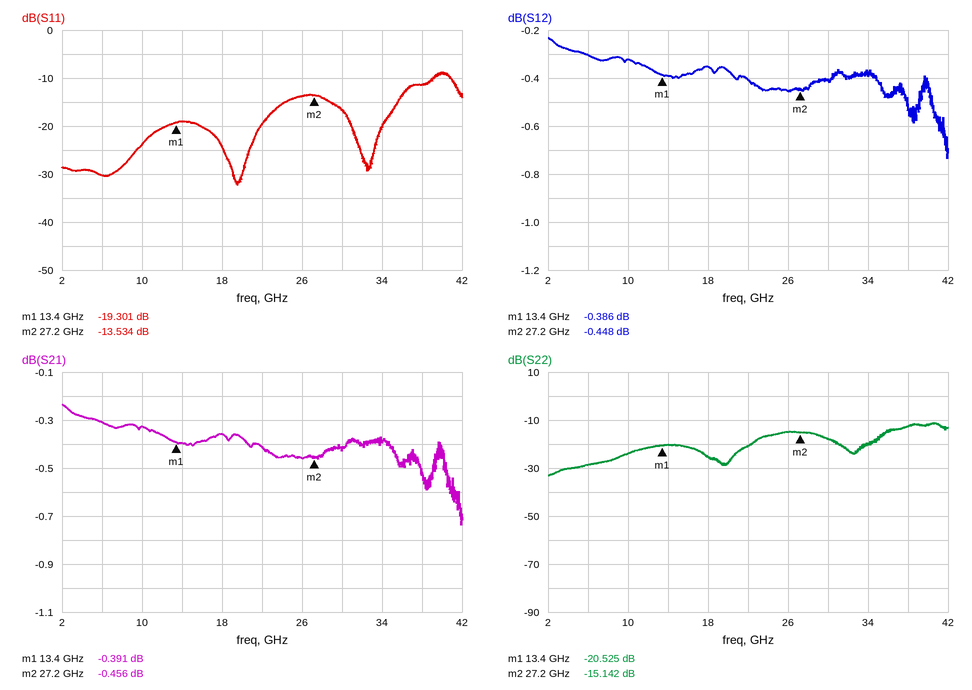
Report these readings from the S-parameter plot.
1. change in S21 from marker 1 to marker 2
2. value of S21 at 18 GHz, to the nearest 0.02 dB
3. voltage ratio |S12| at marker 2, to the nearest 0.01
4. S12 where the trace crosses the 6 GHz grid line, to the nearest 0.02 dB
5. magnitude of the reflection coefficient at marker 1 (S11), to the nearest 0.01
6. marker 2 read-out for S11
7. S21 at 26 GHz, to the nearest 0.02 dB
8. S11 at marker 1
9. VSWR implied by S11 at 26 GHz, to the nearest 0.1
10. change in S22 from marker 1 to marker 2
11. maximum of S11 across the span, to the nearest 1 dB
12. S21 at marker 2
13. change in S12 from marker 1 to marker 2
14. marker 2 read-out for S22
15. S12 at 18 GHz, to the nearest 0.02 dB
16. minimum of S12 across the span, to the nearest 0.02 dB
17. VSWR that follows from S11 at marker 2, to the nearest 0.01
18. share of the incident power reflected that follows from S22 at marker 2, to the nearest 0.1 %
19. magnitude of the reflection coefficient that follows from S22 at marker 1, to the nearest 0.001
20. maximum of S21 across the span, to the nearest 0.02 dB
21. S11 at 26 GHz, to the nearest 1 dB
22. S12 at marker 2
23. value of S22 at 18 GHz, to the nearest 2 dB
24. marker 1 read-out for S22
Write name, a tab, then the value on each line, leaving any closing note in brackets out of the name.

change in S21 from marker 1 to marker 2	-0.065 dB
value of S21 at 18 GHz, to the nearest 0.02 dB	-0.36 dB
voltage ratio |S12| at marker 2, to the nearest 0.01	0.95
S12 where the trace crosses the 6 GHz grid line, to the nearest 0.02 dB	-0.30 dB
magnitude of the reflection coefficient at marker 1 (S11), to the nearest 0.01	0.11
marker 2 read-out for S11	-13.534 dB
S21 at 26 GHz, to the nearest 0.02 dB	-0.46 dB
S11 at marker 1	-19.301 dB
VSWR implied by S11 at 26 GHz, to the nearest 0.1	1.5
change in S22 from marker 1 to marker 2	5.383 dB
maximum of S11 across the span, to the nearest 1 dB	-9 dB
S21 at marker 2	-0.456 dB
change in S12 from marker 1 to marker 2	-0.062 dB
marker 2 read-out for S22	-15.142 dB
S12 at 18 GHz, to the nearest 0.02 dB	-0.36 dB
minimum of S12 across the span, to the nearest 0.02 dB	-0.74 dB
VSWR that follows from S11 at marker 2, to the nearest 0.01	1.53
share of the incident power reflected that follows from S22 at marker 2, to the nearest 0.1 %	3.1 %
magnitude of the reflection coefficient that follows from S22 at marker 1, to the nearest 0.001	0.094
maximum of S21 across the span, to the nearest 0.02 dB	-0.24 dB
S11 at 26 GHz, to the nearest 1 dB	-14 dB
S12 at marker 2	-0.448 dB
value of S22 at 18 GHz, to the nearest 2 dB	-26 dB
marker 1 read-out for S22	-20.525 dB
